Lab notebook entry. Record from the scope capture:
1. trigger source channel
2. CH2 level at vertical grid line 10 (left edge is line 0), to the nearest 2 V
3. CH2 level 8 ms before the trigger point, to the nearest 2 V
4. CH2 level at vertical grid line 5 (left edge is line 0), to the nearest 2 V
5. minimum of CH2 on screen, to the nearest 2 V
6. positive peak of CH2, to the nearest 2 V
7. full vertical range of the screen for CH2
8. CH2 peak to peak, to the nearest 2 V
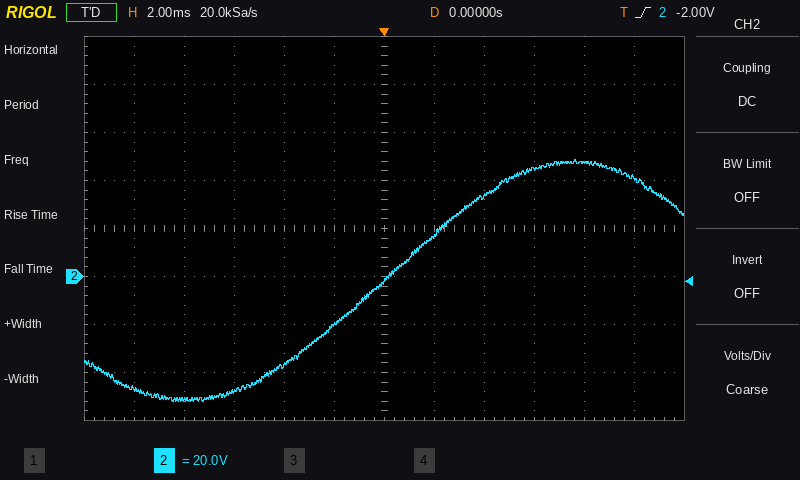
CH2
48 V
-52 V
-20 V
-52 V
48 V
160 V
100 V
